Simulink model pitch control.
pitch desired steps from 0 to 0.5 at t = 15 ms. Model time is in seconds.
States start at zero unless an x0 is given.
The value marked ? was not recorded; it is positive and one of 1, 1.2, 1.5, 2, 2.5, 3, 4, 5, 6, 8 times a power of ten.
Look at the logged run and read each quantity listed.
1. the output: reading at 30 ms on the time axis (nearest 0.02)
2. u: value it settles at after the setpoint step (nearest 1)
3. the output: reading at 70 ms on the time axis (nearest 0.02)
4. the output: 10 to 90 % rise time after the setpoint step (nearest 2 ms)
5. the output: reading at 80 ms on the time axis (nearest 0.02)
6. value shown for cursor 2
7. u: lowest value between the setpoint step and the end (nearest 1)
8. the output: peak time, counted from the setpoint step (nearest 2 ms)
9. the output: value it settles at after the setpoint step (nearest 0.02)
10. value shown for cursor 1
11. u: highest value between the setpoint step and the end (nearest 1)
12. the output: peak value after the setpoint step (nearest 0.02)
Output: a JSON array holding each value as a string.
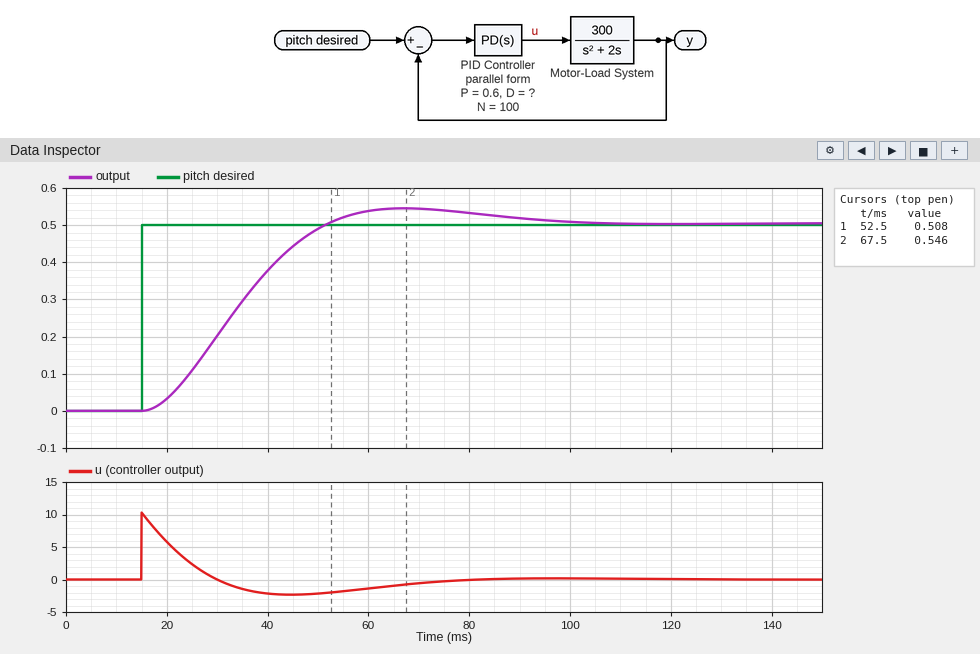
["0.20", "0", "0.54", "24 ms", "0.54", "0.546", "-2", "52 ms", "0.50", "0.508", "10", "0.54"]
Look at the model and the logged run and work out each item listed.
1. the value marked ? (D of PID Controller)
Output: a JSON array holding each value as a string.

["0.2"]
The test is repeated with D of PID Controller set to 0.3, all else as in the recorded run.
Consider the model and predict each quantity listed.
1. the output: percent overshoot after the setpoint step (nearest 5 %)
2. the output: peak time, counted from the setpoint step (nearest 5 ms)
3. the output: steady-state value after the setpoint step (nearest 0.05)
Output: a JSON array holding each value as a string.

["15 %", "40 ms", "0.50"]
